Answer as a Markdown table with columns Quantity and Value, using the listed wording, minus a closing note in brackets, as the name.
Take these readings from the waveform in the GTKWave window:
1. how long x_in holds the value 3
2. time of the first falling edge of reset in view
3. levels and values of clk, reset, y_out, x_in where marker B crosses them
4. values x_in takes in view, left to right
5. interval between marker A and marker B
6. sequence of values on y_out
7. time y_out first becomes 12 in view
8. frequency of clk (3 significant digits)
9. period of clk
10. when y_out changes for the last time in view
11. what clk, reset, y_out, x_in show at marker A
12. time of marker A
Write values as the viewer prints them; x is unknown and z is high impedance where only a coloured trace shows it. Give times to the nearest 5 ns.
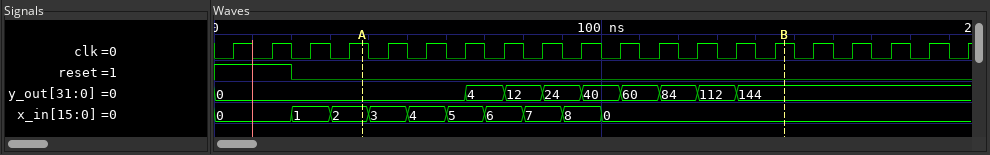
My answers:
| Quantity | Value |
|---|---|
| how long x_in holds the value 3 | 10 ns |
| time of the first falling edge of reset in view | 20 ns |
| levels and values of clk, reset, y_out, x_in where marker B crosses them | clk=1, reset=0, y_out=144, x_in=0 |
| values x_in takes in view, left to right | 0, 1, 2, 3, 4, 5, 6, 7, 8, 0 |
| interval between marker A and marker B | 110 ns |
| sequence of values on y_out | 0, 4, 12, 24, 40, 60, 84, 112, 144 |
| time y_out first becomes 12 in view | 75 ns |
| frequency of clk | 100 MHz |
| period of clk | 10 ns |
| when y_out changes for the last time in view | 135 ns |
| what clk, reset, y_out, x_in show at marker A | clk=1, reset=0, y_out=0, x_in=2 |
| time of marker A | 40 ns |
